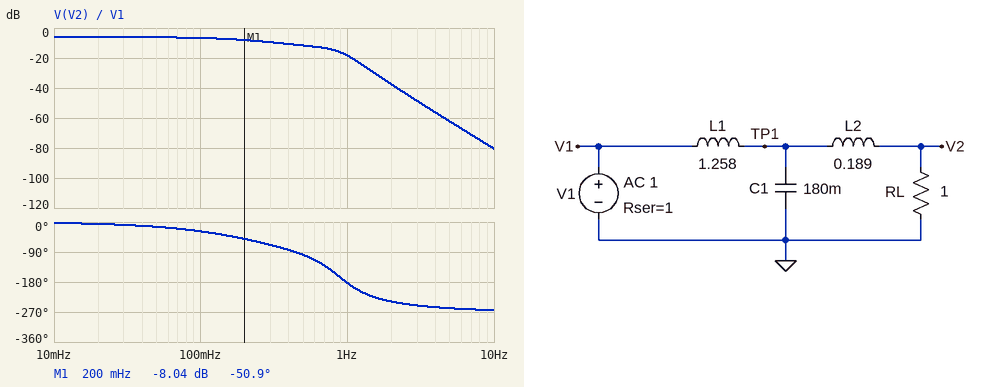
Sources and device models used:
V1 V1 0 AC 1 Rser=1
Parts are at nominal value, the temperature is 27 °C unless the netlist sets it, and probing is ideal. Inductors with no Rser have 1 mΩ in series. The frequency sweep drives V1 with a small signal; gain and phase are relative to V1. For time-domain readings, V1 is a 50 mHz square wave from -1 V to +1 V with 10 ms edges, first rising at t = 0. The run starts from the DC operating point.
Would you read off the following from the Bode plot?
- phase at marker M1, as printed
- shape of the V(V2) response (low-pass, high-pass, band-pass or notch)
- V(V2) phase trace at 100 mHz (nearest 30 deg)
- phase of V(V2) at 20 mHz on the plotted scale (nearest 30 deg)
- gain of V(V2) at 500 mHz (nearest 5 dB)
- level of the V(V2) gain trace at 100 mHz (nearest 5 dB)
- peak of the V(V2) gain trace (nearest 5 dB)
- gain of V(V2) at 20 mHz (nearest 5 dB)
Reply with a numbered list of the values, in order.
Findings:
1. -50.9 deg
2. low-pass
3. -30 deg
4. 0 deg
5. -10 dB
6. -5 dB
7. -5 dB
8. -5 dB
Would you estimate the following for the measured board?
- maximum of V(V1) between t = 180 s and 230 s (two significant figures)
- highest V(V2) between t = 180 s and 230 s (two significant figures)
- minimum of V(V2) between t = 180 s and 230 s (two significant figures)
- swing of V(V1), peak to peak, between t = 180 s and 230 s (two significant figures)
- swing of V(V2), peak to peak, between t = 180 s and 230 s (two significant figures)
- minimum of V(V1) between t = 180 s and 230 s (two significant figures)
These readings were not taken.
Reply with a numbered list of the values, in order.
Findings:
1. 1.5 V
2. 500 mV
3. -500 mV
4. 3.0 V
5. 1.0 V
6. -1.5 V
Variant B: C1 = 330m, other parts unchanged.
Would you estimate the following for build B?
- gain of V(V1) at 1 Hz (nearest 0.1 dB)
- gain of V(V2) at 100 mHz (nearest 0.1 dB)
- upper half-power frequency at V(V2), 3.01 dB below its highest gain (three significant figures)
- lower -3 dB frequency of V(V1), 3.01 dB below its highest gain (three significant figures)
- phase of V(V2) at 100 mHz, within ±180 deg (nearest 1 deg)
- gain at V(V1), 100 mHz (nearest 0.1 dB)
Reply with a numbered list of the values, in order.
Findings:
1. -0.1 dB
2. -6.5 dB
3. 298 mHz
4. 206 mHz
5. -31 deg
6. -4.8 dB
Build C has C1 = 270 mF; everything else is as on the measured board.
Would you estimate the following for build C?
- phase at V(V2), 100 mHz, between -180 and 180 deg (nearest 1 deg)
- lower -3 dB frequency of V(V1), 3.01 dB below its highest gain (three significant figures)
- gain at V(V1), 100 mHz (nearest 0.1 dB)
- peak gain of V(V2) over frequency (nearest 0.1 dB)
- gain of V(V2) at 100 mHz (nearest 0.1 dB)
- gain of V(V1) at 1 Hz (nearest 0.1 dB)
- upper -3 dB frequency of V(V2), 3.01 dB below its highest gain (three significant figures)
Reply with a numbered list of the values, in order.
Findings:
1. -30 deg
2. 194 mHz
3. -4.7 dB
4. -6.0 dB
5. -6.6 dB
6. -0.1 dB
7. 290 mHz
